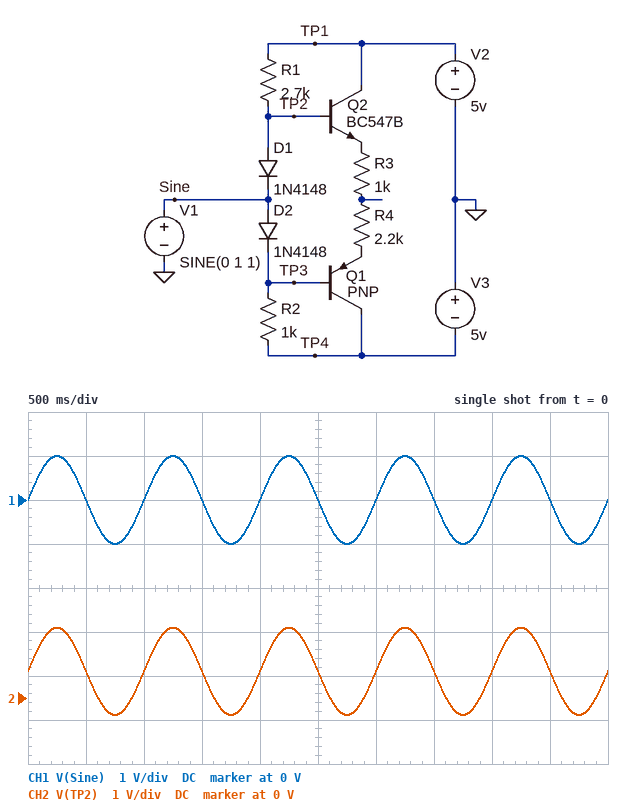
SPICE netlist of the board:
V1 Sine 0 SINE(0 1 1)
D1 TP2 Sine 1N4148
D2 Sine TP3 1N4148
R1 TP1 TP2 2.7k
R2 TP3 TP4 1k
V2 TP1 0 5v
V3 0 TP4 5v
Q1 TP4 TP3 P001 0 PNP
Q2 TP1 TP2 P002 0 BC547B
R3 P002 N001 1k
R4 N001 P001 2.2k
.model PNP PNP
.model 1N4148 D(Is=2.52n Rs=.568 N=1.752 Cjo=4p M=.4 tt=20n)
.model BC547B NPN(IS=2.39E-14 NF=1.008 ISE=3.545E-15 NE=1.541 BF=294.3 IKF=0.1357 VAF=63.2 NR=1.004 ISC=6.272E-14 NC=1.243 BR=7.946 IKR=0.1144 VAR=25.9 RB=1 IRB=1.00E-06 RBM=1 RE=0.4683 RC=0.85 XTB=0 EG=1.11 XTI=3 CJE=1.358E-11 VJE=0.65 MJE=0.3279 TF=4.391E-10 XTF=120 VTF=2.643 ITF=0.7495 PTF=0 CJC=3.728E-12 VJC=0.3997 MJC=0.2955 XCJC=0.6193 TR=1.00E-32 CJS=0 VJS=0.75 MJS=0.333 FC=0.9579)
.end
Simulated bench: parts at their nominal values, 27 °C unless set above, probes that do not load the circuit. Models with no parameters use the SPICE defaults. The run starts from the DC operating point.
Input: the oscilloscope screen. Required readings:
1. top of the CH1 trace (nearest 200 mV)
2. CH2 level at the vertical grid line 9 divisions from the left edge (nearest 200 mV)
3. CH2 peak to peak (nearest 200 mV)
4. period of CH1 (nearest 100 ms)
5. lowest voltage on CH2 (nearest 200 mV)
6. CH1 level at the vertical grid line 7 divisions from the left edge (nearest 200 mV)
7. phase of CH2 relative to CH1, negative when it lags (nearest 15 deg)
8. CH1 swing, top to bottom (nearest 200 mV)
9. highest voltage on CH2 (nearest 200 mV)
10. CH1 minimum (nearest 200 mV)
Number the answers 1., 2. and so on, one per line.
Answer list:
1. 1.0 V
2. 600 mV
3. 2.0 V
4. 1.0 s
5. -400 mV
6. 0 V
7. 0 deg
8. 2.0 V
9. 1.6 V
10. -1.0 V
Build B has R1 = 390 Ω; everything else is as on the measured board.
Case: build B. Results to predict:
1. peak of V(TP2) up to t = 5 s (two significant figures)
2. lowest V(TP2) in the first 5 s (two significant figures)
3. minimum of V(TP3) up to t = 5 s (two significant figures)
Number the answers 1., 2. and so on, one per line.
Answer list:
1. 1.7 V
2. -290 mV
3. -1.6 V
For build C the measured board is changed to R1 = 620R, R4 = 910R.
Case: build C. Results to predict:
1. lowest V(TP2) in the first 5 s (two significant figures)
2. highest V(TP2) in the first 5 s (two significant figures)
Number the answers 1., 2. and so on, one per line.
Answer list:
1. -310 mV
2. 1.7 V
